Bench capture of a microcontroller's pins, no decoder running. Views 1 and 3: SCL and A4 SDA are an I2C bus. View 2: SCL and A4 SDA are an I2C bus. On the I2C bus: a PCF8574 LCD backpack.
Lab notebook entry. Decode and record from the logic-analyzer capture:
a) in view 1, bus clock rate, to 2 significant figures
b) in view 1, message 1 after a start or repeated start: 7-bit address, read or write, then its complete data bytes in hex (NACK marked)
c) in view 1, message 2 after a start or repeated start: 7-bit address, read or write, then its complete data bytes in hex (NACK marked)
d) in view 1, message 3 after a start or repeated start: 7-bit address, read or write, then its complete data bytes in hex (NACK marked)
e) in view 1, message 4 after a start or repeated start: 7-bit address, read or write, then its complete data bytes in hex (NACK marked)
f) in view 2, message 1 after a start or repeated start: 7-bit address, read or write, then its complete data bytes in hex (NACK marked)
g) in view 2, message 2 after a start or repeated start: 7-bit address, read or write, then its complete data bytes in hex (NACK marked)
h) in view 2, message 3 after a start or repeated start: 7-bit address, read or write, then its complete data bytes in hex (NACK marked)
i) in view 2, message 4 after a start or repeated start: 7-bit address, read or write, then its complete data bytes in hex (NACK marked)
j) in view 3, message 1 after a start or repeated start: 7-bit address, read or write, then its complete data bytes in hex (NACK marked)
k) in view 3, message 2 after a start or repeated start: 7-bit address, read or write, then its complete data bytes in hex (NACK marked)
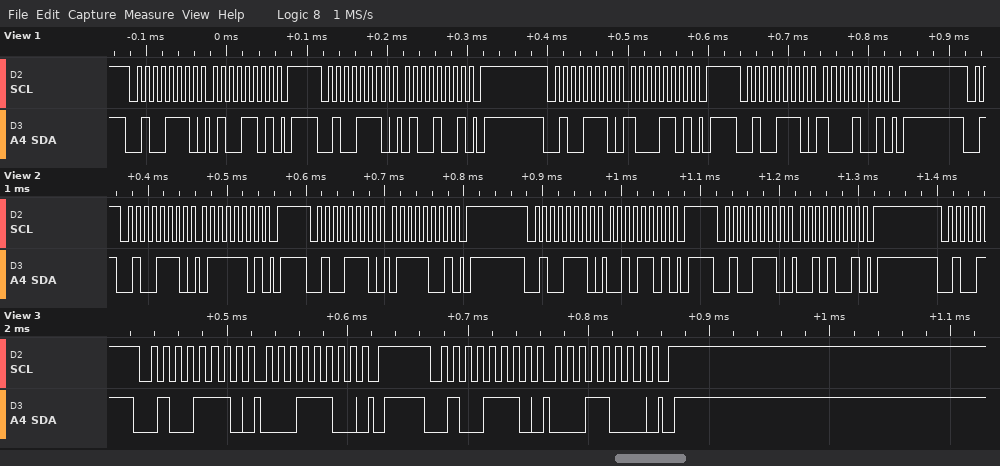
100 kHz
0x27 write: 4D
0x27 write: 49
0x27 write: 8D
0x27 write: 89
0x27 write: 7D
0x27 write: 79
0x27 write: 2D
0x27 write: 29
0x27 write: 1C
0x27 write: 18
